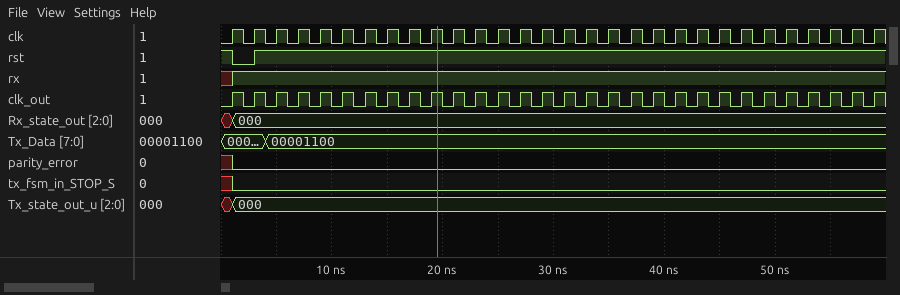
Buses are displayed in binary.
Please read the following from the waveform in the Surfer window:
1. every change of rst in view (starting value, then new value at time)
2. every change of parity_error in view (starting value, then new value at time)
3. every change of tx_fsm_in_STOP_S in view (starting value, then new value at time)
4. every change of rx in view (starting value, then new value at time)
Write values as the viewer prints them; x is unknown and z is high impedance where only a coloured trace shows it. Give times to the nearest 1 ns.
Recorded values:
1, 0 at 1 ns, 1 at 3 ns
x, 0 at 1 ns
x, 0 at 1 ns
x, 1 at 1 ns
